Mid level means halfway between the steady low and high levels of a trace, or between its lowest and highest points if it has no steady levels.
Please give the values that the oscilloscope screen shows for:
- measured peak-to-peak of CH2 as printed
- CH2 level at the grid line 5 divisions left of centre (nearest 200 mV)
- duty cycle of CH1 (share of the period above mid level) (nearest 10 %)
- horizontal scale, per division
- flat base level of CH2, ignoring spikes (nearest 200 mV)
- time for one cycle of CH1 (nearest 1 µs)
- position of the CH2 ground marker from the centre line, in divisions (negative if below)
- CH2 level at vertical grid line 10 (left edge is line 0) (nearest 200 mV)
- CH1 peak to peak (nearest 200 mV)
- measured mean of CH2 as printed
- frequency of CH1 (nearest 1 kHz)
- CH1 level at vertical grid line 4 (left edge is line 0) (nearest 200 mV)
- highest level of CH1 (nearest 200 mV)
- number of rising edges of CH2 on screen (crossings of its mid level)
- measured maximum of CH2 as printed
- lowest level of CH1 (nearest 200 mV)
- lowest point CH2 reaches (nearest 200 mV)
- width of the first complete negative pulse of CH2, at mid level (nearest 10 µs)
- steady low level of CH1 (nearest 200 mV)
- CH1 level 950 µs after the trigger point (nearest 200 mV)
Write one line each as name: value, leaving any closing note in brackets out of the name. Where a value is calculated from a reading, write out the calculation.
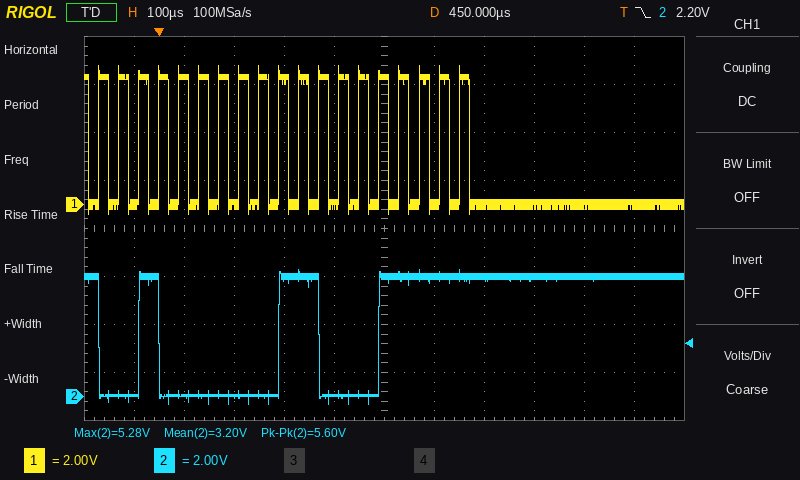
measured peak-to-peak of CH2 as printed: 5.60 V
CH2 level at the grid line 5 divisions left of centre: 0.0 V
duty cycle of CH1 (share of the period above mid level): 50 %
horizontal scale, per division: 100 µs
flat base level of CH2, ignoring spikes: 0.0 V
time for one cycle of CH1: 40 µs
position of the CH2 ground marker from the centre line, in divisions: -3.5 div
CH2 level at vertical grid line 10 (left edge is line 0): 5.0 V
CH1 peak to peak: 5.8 V − (-400 mV) = 6.2 V
measured mean of CH2 as printed: 3.20 V
frequency of CH1: 1 / 40 µs ≈ 25 kHz
CH1 level at vertical grid line 4 (left edge is line 0): 5.2 V
highest level of CH1: 5.8 V
number of rising edges of CH2 on screen: 3
measured maximum of CH2 as printed: 5.28 V
lowest level of CH1: -400 mV
lowest point CH2 reaches: -400 mV
width of the first complete negative pulse of CH2, at mid level: 80 µs
steady low level of CH1: 0.0 V
CH1 level 950 µs after the trigger point: 0.0 V
